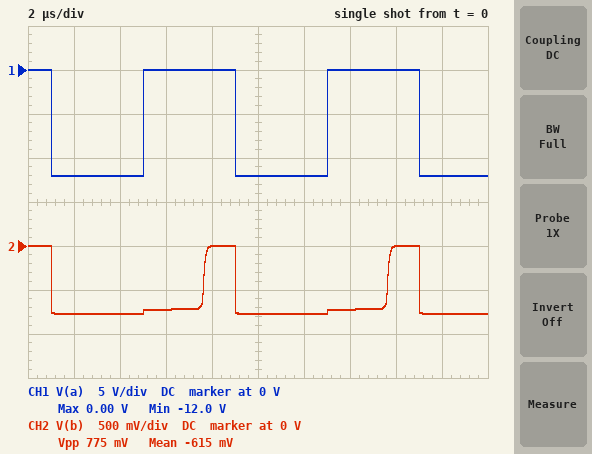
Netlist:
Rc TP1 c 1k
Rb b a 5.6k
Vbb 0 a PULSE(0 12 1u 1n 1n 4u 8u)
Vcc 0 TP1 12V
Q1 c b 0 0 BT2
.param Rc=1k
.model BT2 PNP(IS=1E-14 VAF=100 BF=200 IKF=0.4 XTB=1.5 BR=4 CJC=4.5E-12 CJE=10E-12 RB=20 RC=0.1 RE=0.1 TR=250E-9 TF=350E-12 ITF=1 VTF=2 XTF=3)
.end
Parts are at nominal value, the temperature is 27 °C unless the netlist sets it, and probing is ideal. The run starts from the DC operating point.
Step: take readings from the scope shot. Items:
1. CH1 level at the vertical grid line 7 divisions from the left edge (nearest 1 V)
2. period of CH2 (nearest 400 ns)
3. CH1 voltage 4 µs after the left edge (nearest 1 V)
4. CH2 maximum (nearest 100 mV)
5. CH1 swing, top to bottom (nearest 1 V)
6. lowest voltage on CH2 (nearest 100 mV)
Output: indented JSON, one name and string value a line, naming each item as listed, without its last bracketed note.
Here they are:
{
  "CH1 level at the vertical grid line 7 divisions from the left edge": "0 V",
  "period of CH2": "8.0 µs",
  "CH1 voltage 4 µs after the left edge": "-12 V",
  "CH2 maximum": "0 V",
  "CH1 swing, top to bottom": "12 V",
  "lowest voltage on CH2": "-800 mV"
}
